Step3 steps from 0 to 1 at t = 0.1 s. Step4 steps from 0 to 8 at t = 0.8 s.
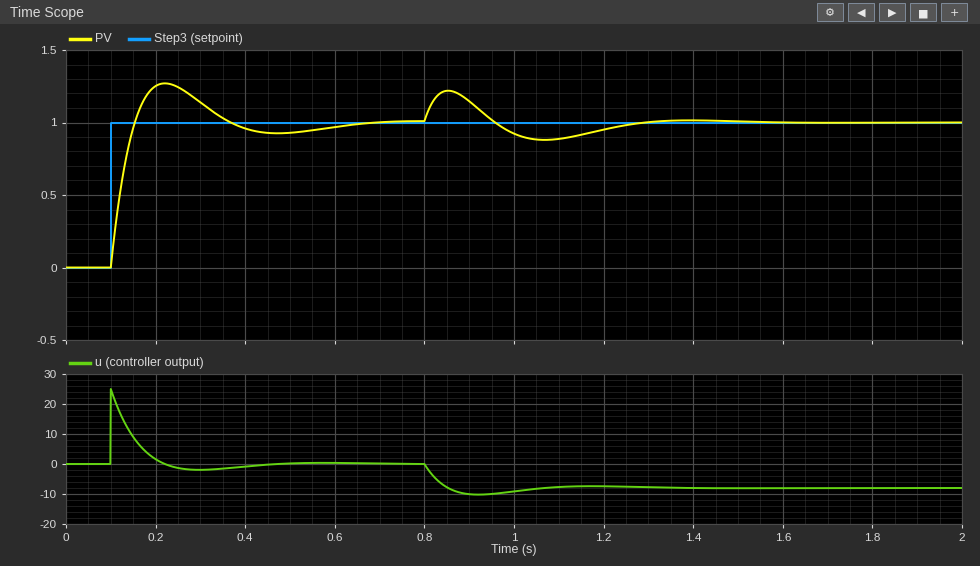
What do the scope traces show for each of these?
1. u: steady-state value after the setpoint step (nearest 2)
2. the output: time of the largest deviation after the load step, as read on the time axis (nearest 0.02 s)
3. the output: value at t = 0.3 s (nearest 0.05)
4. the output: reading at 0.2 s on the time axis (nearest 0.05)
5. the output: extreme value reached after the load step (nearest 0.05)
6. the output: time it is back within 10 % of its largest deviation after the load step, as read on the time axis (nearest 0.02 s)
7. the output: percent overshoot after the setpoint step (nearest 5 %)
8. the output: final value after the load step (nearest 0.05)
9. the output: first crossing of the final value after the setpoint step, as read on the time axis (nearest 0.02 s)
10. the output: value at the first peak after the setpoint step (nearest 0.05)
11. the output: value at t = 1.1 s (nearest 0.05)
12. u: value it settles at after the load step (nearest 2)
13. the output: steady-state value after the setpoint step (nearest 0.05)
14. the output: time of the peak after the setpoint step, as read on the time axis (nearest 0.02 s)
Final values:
0
0.86 s
1.15
1.25
1.20
1.24 s
25 %
1.00
0.16 s
1.25
0.90
-8
1.00
0.22 s
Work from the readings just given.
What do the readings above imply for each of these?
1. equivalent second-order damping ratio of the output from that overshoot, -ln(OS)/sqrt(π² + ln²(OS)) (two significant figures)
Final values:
0.40
